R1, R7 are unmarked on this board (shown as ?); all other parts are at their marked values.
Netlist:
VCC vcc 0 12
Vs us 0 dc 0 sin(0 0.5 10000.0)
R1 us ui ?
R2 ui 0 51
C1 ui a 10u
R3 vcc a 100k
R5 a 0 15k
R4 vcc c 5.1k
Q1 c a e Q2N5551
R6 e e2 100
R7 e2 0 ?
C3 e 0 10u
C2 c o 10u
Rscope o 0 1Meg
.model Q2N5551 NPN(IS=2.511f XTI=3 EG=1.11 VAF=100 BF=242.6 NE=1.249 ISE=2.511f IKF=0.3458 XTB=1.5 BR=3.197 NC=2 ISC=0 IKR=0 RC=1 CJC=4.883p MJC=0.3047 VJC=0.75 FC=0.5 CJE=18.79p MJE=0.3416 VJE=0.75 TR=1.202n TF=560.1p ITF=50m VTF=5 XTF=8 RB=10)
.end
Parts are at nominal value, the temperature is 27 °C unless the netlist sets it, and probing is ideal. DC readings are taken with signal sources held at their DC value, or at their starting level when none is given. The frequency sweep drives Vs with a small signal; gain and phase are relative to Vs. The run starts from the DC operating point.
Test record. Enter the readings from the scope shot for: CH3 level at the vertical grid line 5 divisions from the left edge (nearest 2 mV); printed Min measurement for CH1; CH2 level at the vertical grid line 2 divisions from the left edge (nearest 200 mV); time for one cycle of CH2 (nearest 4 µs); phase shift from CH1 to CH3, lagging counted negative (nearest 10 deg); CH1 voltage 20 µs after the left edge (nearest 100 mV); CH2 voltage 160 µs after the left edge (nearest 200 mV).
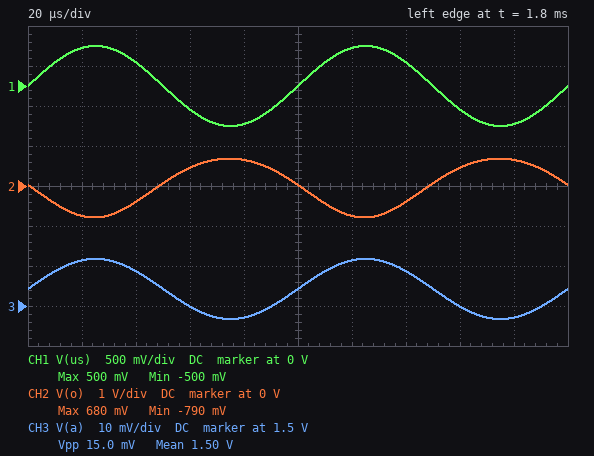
1.504 V
-500 mV
-400 mV
100 µs
0 deg
500 mV
400 mV
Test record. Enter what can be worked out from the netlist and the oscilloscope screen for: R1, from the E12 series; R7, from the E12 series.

3.3 kΩ
1.5 kΩ
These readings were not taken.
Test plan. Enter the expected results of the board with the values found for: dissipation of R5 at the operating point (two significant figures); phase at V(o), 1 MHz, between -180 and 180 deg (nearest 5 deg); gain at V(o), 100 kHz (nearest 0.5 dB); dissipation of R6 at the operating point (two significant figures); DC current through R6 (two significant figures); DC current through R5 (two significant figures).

150 µW
170 deg
3.5 dB
27 µW
520 µA
100 µA
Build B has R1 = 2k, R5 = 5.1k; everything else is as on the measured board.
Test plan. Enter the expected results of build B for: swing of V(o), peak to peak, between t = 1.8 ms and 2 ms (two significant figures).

46 mV
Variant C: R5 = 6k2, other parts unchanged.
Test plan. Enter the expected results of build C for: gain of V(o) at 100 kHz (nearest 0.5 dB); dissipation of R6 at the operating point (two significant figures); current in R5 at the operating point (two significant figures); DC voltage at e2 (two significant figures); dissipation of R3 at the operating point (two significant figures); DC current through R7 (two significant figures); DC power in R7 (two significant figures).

-16.0 dB
280 nW
110 µA
80 mV
1.3 mW
53 µA
4.2 µW
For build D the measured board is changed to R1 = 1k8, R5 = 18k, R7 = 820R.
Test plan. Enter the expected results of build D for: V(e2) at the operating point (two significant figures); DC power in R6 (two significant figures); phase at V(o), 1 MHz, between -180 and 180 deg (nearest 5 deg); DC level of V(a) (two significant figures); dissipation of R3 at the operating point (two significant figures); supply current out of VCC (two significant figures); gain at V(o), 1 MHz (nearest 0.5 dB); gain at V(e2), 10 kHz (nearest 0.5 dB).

890 mV
120 µW
165 deg
1.7 V
1.1 mW
1.2 mA
14.5 dB
-56.5 dB
